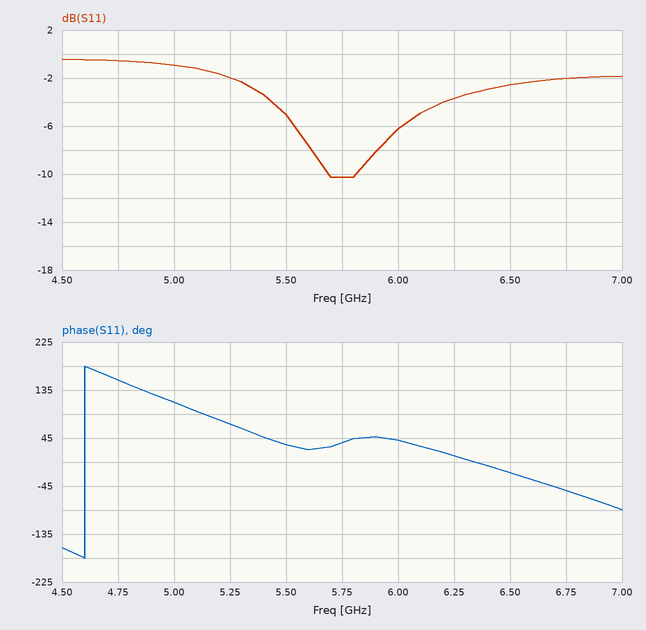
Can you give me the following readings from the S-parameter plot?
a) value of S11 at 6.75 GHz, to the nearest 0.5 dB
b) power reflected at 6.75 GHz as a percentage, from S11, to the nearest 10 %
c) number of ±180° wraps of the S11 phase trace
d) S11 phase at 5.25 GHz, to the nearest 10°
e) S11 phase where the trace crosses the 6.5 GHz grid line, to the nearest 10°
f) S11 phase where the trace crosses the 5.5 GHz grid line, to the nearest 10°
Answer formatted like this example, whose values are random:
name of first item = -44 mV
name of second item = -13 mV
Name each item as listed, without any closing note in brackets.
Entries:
value of S11 at 6.75 GHz, to the nearest 0.5 dB = -2.0 dB
power reflected at 6.75 GHz as a percentage, from S11, to the nearest 10 % = 60 %
number of ±180° wraps of the S11 phase trace = 1
S11 phase at 5.25 GHz, to the nearest 10° = 70°
S11 phase where the trace crosses the 6.5 GHz grid line, to the nearest 10° = -20°
S11 phase where the trace crosses the 5.5 GHz grid line, to the nearest 10° = 30°
